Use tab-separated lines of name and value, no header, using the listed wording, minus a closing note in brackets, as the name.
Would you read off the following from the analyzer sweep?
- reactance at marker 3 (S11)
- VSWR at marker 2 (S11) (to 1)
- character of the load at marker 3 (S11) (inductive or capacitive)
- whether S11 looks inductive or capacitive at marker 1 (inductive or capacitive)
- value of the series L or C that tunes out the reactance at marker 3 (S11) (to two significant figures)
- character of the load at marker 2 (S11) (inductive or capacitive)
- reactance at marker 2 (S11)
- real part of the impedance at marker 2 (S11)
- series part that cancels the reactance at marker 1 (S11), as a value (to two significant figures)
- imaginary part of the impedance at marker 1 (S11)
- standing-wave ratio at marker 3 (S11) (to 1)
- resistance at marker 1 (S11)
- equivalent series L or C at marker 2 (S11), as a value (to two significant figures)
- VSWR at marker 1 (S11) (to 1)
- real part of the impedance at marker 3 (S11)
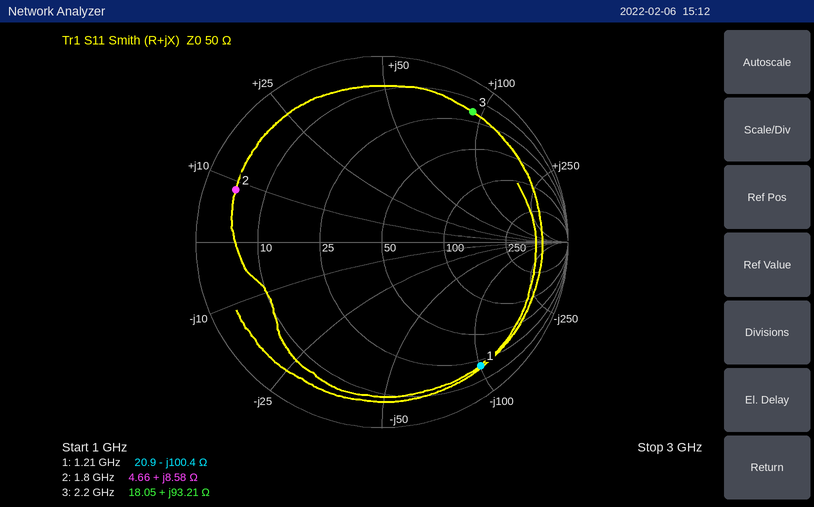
reactance at marker 3	+93.21 Ω
VSWR at marker 2 (S11)	11
character of the load at marker 3 (S11)	inductive
whether S11 looks inductive or capacitive at marker 1	capacitive
value of the series L or C that tunes out the reactance at marker 3 (S11)	780 fF
character of the load at marker 2 (S11)	inductive
reactance at marker 2	+8.58 Ω
real part of the impedance at marker 2	4.66 Ω
series part that cancels the reactance at marker 1 (S11), as a value	13 nH
imaginary part of the impedance at marker 1	-100.4 Ω
standing-wave ratio at marker 3 (S11)	13
resistance at marker 1	20.9 Ω
equivalent series L or C at marker 2 (S11), as a value	760 pH
VSWR at marker 1 (S11)	12
real part of the impedance at marker 3	18.05 Ω
